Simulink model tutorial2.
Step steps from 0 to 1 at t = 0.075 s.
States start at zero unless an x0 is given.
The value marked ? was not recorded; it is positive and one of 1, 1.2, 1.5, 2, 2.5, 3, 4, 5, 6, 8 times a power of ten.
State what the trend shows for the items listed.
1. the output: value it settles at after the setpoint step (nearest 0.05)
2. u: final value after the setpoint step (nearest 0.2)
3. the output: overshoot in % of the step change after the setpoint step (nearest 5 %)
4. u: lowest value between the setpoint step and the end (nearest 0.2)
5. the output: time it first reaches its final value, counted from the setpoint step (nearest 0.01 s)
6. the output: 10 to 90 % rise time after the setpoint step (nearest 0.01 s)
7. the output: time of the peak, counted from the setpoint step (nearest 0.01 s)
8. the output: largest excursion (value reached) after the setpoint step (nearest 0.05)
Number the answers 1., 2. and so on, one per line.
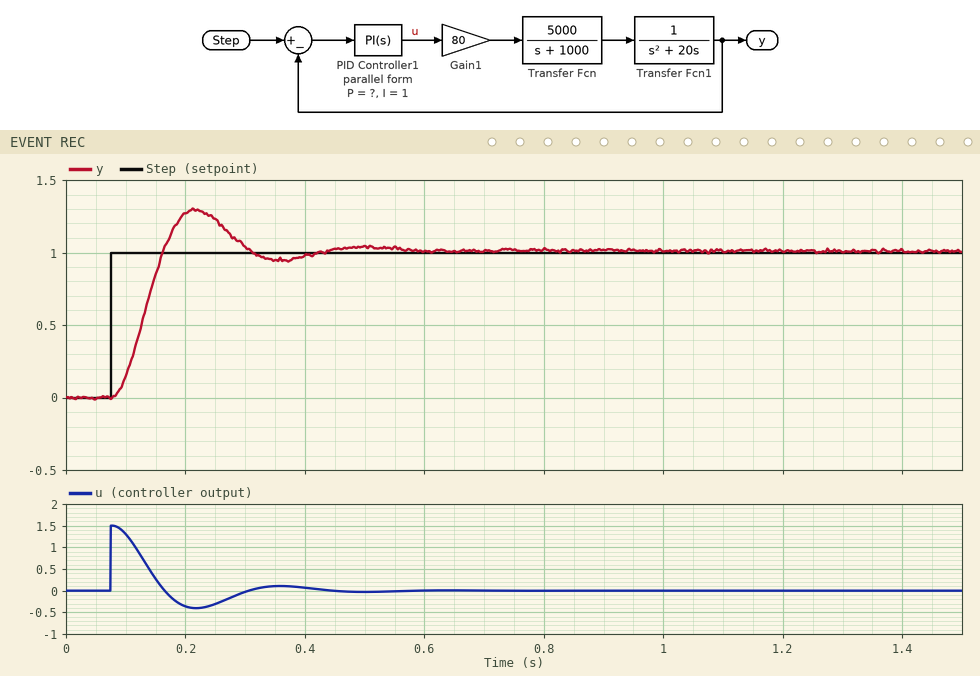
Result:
1. 1.00
2. 0.0
3. 30 %
4. -0.4
5. 0.09 s
6. 0.06 s
7. 0.14 s
8. 1.30
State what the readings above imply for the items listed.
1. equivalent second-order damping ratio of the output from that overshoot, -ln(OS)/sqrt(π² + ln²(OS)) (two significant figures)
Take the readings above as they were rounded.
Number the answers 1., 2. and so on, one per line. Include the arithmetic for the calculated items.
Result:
1. ln(0.3) = -1.204; 1.204 / sqrt(9.870 + 1.450) = 0.36
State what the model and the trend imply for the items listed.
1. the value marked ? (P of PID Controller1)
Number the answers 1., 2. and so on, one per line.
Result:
1. 1.5
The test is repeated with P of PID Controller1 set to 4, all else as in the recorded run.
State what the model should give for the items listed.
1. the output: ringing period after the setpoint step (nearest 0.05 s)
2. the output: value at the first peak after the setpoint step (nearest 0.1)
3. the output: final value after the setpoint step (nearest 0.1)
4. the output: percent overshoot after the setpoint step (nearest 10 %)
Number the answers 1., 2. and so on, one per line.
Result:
1. 0.15 s
2. 1.5
3. 1.0
4. 50 %
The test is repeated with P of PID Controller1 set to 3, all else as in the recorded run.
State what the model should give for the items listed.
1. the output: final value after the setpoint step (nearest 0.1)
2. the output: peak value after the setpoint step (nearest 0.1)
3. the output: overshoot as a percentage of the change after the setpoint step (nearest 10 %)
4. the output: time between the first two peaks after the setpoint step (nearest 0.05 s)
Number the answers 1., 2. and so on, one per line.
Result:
1. 1.0
2. 1.4
3. 40 %
4. 0.20 s
